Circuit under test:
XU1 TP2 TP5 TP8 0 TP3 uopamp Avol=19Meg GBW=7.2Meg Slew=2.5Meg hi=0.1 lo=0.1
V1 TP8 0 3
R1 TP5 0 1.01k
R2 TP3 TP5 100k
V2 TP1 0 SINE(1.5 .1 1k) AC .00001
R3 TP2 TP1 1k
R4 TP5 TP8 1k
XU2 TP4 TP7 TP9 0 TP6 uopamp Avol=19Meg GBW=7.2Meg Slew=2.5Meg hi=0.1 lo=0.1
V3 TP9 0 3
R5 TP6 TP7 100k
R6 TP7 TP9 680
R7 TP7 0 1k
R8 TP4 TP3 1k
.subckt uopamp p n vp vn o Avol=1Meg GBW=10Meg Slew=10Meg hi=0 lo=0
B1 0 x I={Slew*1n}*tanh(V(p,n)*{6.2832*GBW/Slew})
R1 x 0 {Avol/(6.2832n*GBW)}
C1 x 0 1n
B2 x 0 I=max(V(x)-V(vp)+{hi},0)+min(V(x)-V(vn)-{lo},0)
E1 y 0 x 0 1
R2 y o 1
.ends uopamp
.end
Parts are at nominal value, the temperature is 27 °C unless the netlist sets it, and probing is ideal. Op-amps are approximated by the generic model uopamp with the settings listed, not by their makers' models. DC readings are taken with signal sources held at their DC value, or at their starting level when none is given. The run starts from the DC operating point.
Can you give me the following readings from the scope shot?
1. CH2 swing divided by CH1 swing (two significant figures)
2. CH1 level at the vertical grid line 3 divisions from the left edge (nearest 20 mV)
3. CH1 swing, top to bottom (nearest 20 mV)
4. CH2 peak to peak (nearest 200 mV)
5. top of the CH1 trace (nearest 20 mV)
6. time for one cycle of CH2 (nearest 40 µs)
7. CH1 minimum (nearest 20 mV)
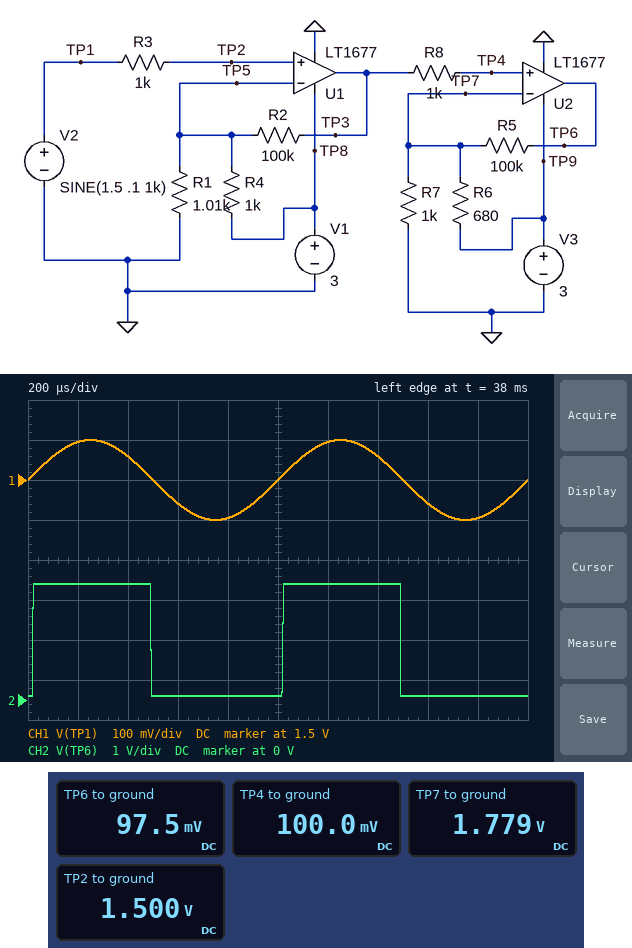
14
1.44 V
200 mV
2.8 V
1.60 V
1.00 ms
1.40 V
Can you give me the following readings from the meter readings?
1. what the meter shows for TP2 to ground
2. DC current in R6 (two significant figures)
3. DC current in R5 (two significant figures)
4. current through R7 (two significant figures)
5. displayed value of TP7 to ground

1.500 V
1.8 mA
17 µA
1.8 mA
1.779 V
